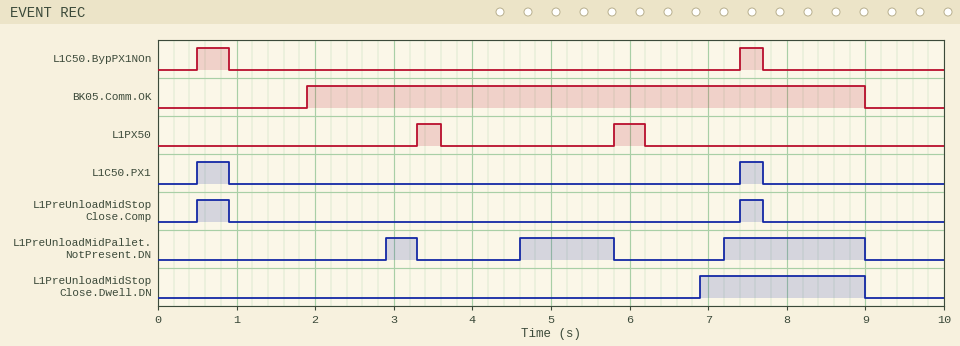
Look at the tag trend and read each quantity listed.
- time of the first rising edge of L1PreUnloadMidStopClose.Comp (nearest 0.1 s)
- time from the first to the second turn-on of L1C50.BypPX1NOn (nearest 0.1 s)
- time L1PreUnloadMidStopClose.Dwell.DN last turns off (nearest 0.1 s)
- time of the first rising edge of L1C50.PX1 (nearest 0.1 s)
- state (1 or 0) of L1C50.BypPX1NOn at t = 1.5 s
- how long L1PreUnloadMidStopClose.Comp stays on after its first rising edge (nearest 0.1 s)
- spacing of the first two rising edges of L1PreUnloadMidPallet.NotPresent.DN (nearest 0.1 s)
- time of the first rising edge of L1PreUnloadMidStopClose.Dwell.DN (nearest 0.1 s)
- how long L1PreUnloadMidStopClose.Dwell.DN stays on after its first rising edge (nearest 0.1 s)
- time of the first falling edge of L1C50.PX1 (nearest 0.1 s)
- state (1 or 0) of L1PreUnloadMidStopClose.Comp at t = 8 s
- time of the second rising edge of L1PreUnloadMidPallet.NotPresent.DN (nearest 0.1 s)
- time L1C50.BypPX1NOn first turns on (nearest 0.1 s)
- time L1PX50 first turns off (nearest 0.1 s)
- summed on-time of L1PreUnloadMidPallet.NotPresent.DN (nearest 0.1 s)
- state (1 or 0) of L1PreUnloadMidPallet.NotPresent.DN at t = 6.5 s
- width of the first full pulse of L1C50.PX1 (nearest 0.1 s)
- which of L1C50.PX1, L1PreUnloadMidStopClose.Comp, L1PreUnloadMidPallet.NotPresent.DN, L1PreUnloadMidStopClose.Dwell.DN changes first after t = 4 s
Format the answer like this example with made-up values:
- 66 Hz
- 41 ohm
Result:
- 0.5 s
- 6.9 s
- 9.0 s
- 0.5 s
- 0
- 0.4 s
- 1.7 s
- 6.9 s
- 2.1 s
- 0.9 s
- 0
- 4.6 s
- 0.5 s
- 3.6 s
- 3.4 s
- 0
- 0.4 s
- L1PreUnloadMidPallet.NotPresent.DN
